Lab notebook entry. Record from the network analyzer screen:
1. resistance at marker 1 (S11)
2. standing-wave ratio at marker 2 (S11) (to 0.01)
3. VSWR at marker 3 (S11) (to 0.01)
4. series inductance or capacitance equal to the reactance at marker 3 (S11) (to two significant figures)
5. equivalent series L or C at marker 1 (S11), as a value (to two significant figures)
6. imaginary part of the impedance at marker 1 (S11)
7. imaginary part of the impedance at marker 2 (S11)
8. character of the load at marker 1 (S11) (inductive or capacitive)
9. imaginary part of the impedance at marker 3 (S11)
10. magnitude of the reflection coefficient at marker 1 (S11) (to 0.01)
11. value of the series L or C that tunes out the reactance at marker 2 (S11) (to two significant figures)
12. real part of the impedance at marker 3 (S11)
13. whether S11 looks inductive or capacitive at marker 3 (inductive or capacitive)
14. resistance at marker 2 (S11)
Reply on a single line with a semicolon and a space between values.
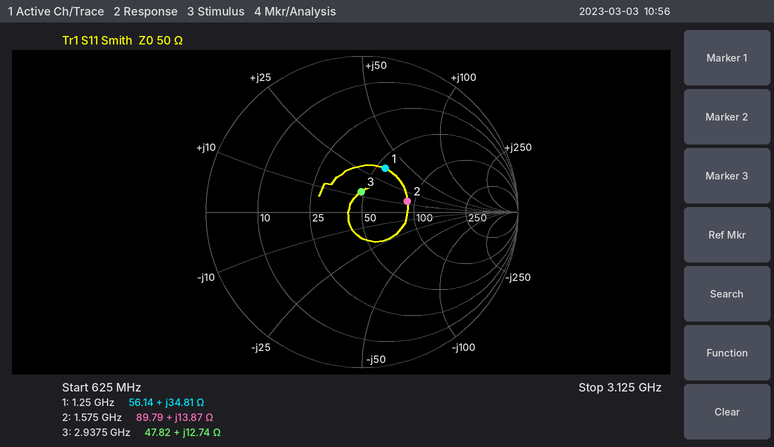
56.14 Ω; 1.86; 1.30; 690 pH; 4.4 nH; +34.81 Ω; +13.87 Ω; inductive; +12.74 Ω; 0.32; 7.3 pF; 47.82 Ω; inductive; 89.79 Ω
